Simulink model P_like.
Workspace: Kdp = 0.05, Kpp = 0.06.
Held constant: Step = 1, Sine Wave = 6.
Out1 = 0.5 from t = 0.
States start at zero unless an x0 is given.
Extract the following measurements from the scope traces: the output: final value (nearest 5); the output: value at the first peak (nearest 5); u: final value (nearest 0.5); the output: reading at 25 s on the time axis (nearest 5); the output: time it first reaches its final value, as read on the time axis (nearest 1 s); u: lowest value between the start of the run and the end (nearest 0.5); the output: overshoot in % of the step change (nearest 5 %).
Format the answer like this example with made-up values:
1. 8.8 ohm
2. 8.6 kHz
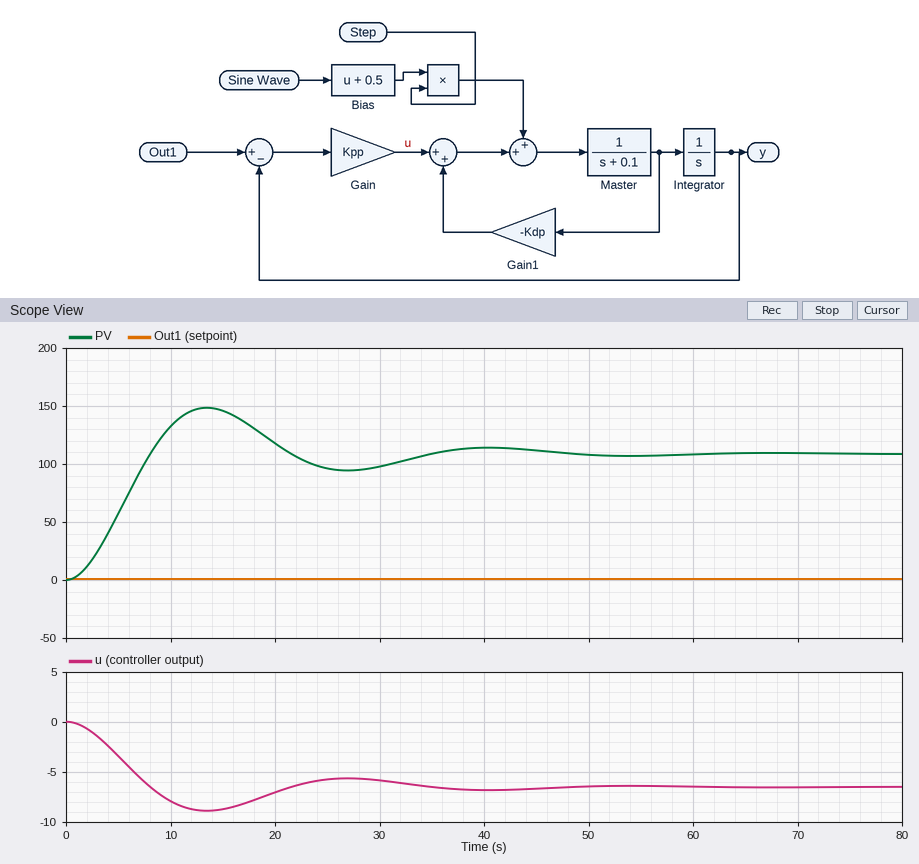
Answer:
1. 110
2. 150
3. -6.5
4. 95
5. 8 s
6. -9.0
7. 35 %
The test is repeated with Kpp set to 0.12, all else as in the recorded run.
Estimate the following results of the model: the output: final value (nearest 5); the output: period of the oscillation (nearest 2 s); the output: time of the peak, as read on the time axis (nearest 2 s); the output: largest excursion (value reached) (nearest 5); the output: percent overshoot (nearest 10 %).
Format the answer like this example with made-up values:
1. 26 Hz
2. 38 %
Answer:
1. 55
2. 18 s
3. 10 s
4. 80
5. 50 %
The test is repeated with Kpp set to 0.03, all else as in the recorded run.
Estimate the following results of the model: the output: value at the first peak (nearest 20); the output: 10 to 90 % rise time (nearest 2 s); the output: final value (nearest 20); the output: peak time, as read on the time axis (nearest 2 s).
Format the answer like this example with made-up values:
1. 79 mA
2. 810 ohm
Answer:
1. 260
2. 8 s
3. 220
4. 20 s
